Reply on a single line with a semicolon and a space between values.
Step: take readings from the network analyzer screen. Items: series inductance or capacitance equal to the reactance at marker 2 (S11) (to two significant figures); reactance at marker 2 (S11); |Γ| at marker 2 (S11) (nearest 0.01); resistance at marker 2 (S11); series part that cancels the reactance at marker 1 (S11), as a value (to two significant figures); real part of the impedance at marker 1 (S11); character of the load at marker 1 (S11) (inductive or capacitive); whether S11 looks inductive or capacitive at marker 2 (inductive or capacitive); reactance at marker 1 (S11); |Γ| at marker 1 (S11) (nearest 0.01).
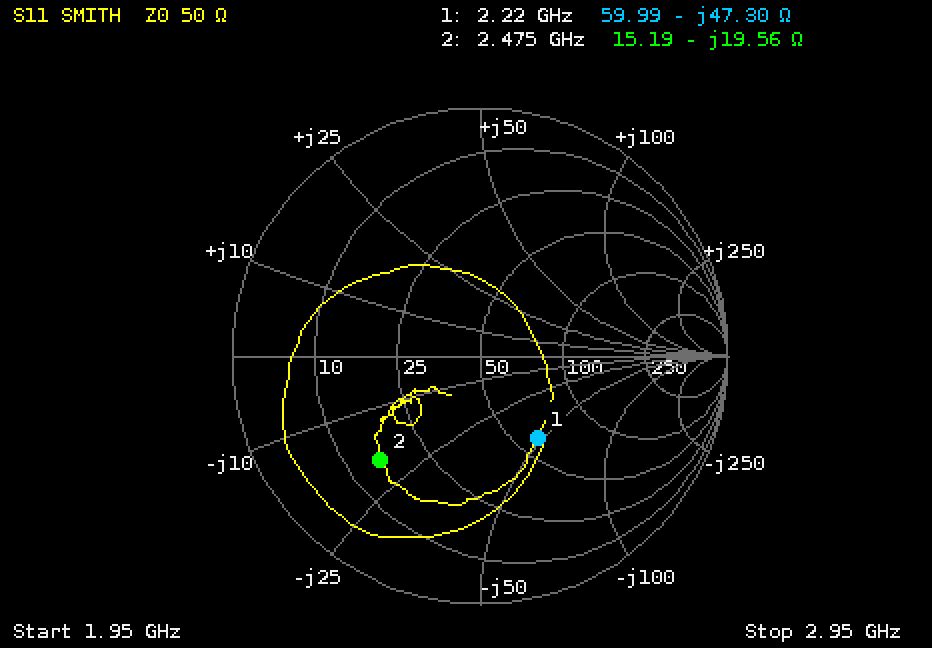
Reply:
3.3 pF; -19.56 Ω; 0.59; 15.19 Ω; 3.4 nH; 59.99 Ω; capacitive; capacitive; -47.30 Ω; 0.40
